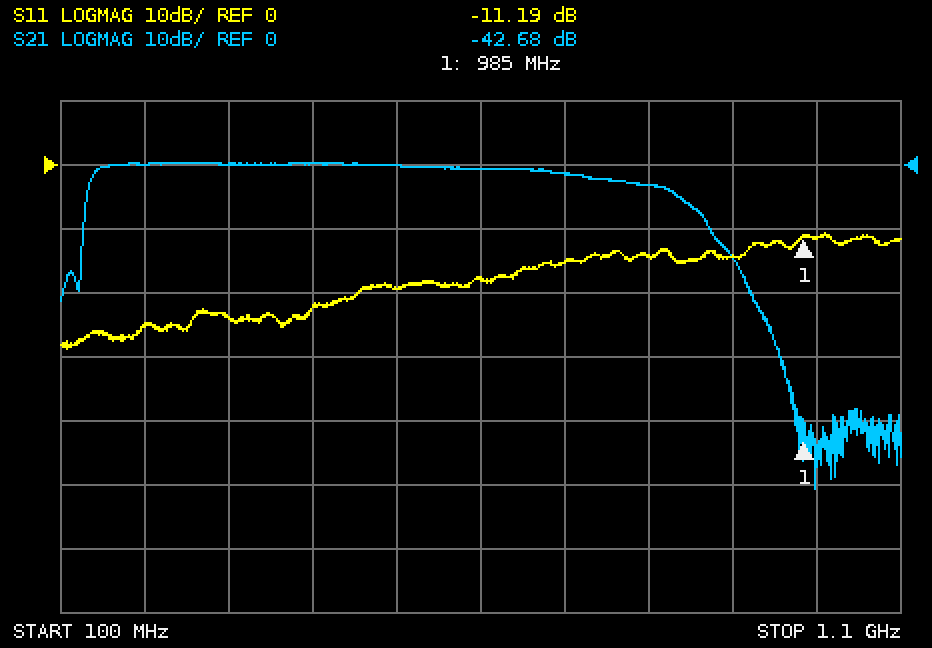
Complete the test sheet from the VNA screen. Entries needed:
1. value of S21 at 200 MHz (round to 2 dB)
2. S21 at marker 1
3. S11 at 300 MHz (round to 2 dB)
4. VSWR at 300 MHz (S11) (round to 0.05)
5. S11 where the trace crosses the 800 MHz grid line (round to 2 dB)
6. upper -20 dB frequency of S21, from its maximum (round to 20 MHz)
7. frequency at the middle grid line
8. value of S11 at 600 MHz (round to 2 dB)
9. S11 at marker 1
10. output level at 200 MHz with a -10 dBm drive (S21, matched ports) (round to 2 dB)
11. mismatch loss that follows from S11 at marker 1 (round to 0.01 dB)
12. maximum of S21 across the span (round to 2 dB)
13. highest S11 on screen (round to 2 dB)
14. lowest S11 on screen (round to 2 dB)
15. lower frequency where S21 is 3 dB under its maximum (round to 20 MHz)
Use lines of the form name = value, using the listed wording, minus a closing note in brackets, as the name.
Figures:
value of S21 at 200 MHz = 0 dB
S21 at marker 1 = -42.68 dB
S11 at 300 MHz = -24 dB
VSWR at 300 MHz (S11) = 1.15
S11 where the trace crosses the 800 MHz grid line = -14 dB
upper -20 dB frequency of S21, from its maximum = 920 MHz
frequency at the middle grid line = 600 MHz
value of S11 at 600 MHz = -18 dB
S11 at marker 1 = -11.19 dB
output level at 200 MHz with a -10 dBm drive (S21, matched ports) = -10 dBm
mismatch loss that follows from S11 at marker 1 = 0.34 dB
maximum of S21 across the span = 0 dB
highest S11 on screen = -10 dB
lowest S11 on screen = -28 dB
lower frequency where S21 is 3 dB under its maximum = 140 MHz
